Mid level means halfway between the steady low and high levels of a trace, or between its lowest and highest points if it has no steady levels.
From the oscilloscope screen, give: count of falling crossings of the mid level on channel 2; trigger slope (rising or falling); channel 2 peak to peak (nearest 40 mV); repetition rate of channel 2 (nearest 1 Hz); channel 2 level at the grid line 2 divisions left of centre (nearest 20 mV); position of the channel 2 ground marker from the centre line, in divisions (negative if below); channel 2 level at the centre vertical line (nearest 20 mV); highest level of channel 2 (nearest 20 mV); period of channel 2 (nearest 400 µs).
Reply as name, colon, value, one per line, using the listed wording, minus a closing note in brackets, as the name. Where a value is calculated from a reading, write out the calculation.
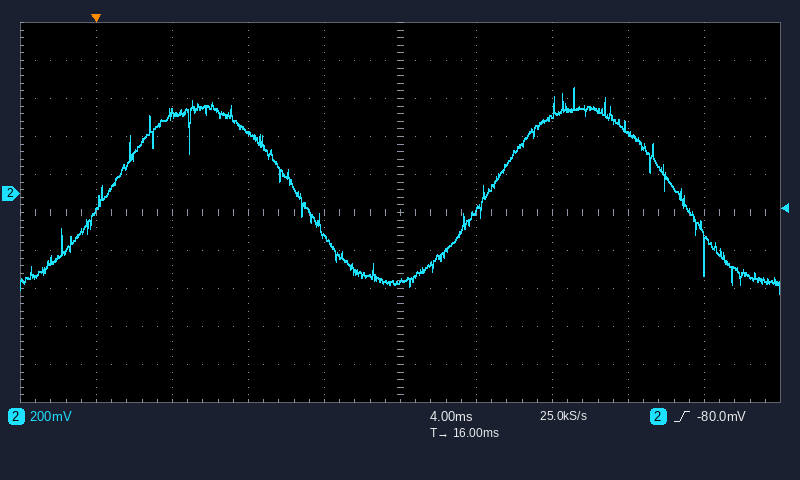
count of falling crossings of the mid level on channel 2: 2
trigger slope: rising
channel 2 peak to peak: 1.08 V
repetition rate of channel 2: 1 / 20.0 ms ≈ 50 Hz
channel 2 level at the grid line 2 divisions left of centre: 320 mV
position of the channel 2 ground marker from the centre line, in divisions: +0.5 div
channel 2 level at the centre vertical line: -460 mV
highest level of channel 2: 560 mV
period of channel 2: 20.0 ms
